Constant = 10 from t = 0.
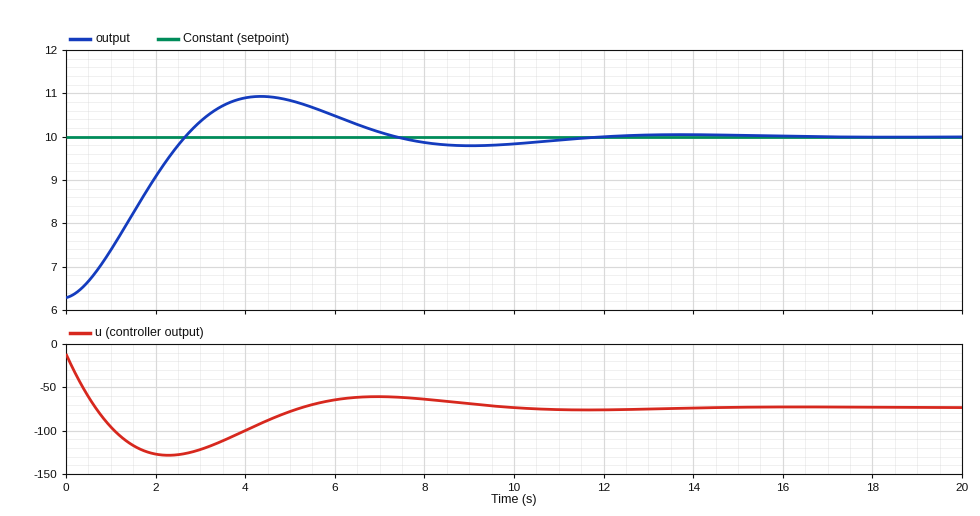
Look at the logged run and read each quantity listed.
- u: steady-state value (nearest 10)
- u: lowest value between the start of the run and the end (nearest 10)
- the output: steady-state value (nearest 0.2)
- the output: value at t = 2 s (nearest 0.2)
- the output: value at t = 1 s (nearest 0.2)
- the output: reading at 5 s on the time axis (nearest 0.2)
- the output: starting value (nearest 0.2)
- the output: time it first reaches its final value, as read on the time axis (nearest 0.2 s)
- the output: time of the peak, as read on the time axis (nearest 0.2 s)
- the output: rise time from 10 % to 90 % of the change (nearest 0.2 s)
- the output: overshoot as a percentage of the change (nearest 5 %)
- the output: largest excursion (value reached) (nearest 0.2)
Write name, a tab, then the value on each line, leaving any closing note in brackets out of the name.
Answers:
u: steady-state value	-70
u: lowest value between the start of the run and the end	-130
the output: steady-state value	10.0
the output: value at t = 2 s	9.0
the output: value at t = 1 s	7.4
the output: reading at 5 s on the time axis	10.8
the output: starting value	6.2
the output: time it first reaches its final value, as read on the time axis	2.6 s
the output: time of the peak, as read on the time axis	4.4 s
the output: rise time from 10 % to 90 % of the change	1.8 s
the output: overshoot as a percentage of the change	25 %
the output: largest excursion (value reached)	11.0
